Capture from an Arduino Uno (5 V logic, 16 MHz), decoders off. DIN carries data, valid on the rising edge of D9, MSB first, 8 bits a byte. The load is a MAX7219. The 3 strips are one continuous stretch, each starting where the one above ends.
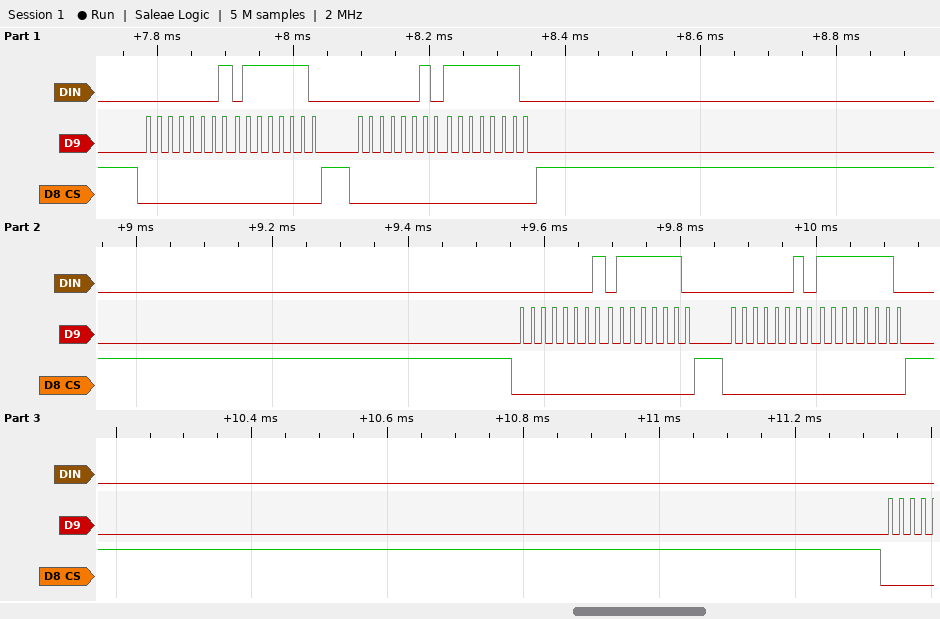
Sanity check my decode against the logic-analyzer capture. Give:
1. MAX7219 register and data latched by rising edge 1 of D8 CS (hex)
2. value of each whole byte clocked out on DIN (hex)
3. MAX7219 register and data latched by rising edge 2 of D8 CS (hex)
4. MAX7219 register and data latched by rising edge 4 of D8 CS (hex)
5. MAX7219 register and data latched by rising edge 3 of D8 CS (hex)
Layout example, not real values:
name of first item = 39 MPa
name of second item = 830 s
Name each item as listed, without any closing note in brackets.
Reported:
MAX7219 register and data latched by rising edge 1 of D8 CS = register 0x1, data 0x7E
value of each whole byte clocked out on DIN = 0x01 0x7E 0x02 0xFE 0x01 0x7E 0x02 0xFE
MAX7219 register and data latched by rising edge 2 of D8 CS = register 0x2, data 0xFE
MAX7219 register and data latched by rising edge 4 of D8 CS = register 0x2, data 0xFE
MAX7219 register and data latched by rising edge 3 of D8 CS = register 0x1, data 0x7E
